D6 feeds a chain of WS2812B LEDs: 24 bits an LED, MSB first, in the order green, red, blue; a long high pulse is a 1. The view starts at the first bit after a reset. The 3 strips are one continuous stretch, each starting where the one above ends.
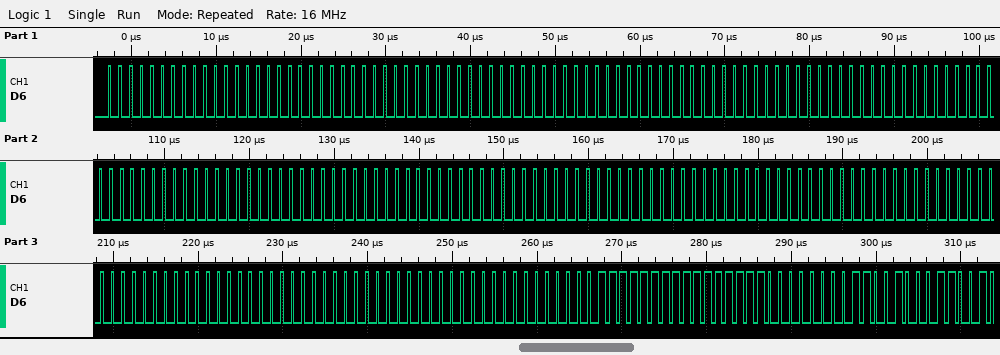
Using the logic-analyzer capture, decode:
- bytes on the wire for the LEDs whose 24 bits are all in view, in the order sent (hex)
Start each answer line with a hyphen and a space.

- 00 00 00 00 00 00 00 00 00 00 00 00 00 00 00 00 00 00 00 00 00 00 00 00 00 00 00 FF FF 00
